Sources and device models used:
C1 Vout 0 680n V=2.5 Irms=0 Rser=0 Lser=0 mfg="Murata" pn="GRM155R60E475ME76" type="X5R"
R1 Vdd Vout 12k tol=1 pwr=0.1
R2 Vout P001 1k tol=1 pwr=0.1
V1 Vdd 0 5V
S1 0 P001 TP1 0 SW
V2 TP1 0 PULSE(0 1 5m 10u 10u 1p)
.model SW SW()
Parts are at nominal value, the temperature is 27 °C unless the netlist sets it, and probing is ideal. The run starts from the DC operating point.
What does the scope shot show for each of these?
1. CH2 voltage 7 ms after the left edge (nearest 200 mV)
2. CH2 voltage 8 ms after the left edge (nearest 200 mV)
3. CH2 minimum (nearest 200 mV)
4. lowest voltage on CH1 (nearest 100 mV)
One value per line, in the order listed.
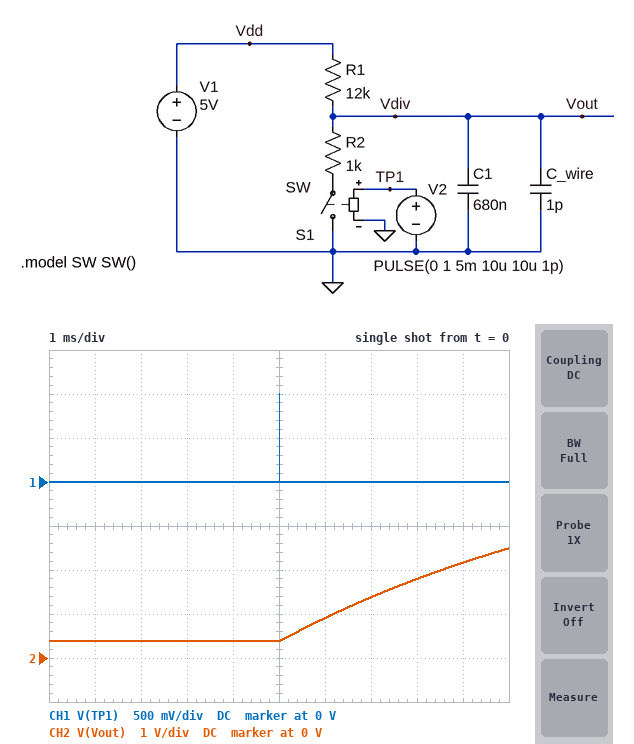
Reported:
1.4 V
1.8 V
400 mV
0 V
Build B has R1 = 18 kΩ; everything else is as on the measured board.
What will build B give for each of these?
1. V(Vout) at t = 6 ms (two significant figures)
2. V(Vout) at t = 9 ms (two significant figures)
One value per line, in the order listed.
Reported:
630 mV
1.6 V
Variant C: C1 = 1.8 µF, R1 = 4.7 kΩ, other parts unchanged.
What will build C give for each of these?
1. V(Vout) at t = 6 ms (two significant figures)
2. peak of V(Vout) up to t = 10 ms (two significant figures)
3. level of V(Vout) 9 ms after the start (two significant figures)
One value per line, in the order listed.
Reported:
1.3 V
2.7 V
2.4 V
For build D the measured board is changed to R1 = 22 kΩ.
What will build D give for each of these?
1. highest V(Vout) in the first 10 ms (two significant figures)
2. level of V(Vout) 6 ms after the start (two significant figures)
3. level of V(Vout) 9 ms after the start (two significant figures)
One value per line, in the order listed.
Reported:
1.6 V
520 mV
1.3 V
